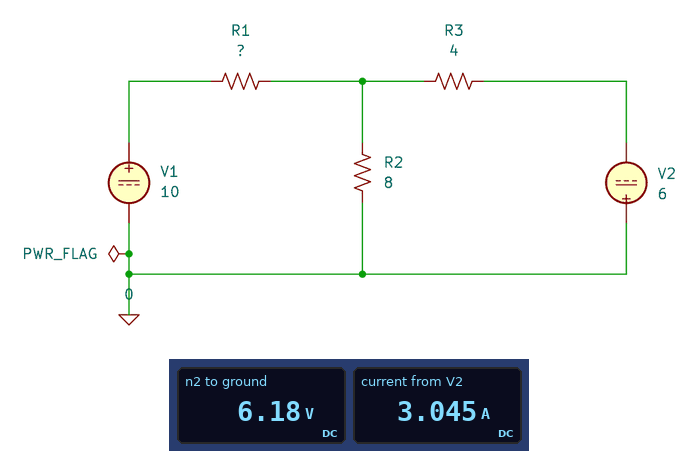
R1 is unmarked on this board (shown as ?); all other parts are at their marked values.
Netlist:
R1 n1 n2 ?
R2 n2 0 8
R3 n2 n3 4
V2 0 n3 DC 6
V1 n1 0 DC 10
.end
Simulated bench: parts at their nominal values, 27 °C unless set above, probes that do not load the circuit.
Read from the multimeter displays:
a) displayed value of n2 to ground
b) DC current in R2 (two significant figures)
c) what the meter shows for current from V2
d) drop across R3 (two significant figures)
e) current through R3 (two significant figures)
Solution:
6.18 V
770 mA
3.045 A
12 V
3.0 A
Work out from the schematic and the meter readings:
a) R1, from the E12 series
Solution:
1 Ω
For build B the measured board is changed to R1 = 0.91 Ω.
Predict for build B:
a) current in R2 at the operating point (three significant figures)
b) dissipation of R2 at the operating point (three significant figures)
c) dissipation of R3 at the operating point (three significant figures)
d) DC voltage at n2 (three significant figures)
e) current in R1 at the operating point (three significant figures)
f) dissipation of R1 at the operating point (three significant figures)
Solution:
805 mA
5.18 W
38.7 W
6.44 V
3.91 A
13.9 W
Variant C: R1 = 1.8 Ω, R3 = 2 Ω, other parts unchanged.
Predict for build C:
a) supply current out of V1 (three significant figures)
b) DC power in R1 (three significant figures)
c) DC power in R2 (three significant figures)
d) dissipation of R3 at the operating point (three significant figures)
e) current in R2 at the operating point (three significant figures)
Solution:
4.35 A
34.1 W
586 mW
33.3 W
271 mA
